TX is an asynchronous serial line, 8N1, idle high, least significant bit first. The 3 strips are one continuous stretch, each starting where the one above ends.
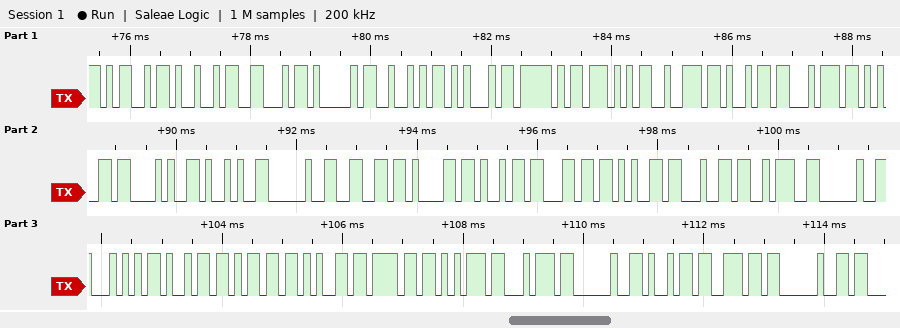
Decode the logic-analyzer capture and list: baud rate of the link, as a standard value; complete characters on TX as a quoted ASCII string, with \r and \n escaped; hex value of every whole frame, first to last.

9600 baud
"MIFARE_Write() failed: Timeout in "
4D 49 46 41 52 45 5F 57 72 69 74 65 28 29 20 66 61 69 6C 65 64 3A 20 54 69 6D 65 6F 75 74 20 69 6E 20
